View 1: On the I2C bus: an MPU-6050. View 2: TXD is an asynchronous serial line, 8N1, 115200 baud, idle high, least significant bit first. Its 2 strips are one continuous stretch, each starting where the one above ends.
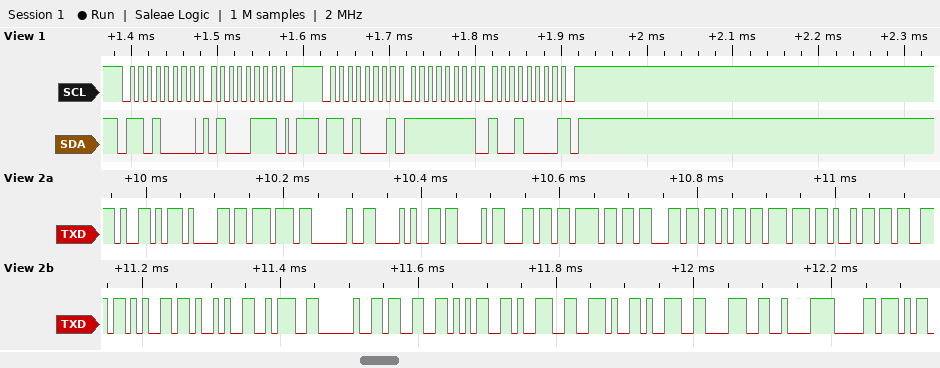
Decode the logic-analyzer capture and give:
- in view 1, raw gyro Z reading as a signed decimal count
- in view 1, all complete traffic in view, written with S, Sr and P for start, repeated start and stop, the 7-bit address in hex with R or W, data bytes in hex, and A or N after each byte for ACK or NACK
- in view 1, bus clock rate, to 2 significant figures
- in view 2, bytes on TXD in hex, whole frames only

-112
S 68W A 47 A P S 68R A FF A 90 N P
100 kHz
59 61 77 20 28 43 6C 6F 63 6B 77 69 73 65 29 3A 20 33 35 39 2E 39 38 C2 B0
